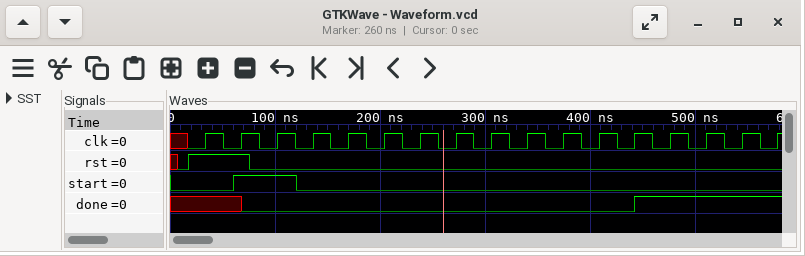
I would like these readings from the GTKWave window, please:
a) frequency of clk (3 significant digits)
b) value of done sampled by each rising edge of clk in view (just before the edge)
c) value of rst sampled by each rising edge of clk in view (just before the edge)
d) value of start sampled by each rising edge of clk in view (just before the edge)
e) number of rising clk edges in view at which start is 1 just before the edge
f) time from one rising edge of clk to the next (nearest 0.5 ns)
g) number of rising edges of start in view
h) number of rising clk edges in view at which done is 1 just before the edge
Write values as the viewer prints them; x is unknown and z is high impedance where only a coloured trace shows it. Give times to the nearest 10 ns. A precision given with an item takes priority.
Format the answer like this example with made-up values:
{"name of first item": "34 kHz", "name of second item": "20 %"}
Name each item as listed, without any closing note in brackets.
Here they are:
{"frequency of clk": "29.4 MHz", "value of done sampled by each rising edge of clk in view": "x x 0 0 0 0 0 0 0 0 0 0 0 1 1 1 1", "value of rst sampled by each rising edge of clk in view": "1 1 0 0 0 0 0 0 0 0 0 0 0 0 0 0 0", "value of start sampled by each rising edge of clk in view": "0 1 1 0 0 0 0 0 0 0 0 0 0 0 0 0 0", "number of rising clk edges in view at which start is 1 just before the edge": "2", "time from one rising edge of clk to the next": "34 ns", "number of rising edges of start in view": "1", "number of rising clk edges in view at which done is 1 just before the edge": "4"}
